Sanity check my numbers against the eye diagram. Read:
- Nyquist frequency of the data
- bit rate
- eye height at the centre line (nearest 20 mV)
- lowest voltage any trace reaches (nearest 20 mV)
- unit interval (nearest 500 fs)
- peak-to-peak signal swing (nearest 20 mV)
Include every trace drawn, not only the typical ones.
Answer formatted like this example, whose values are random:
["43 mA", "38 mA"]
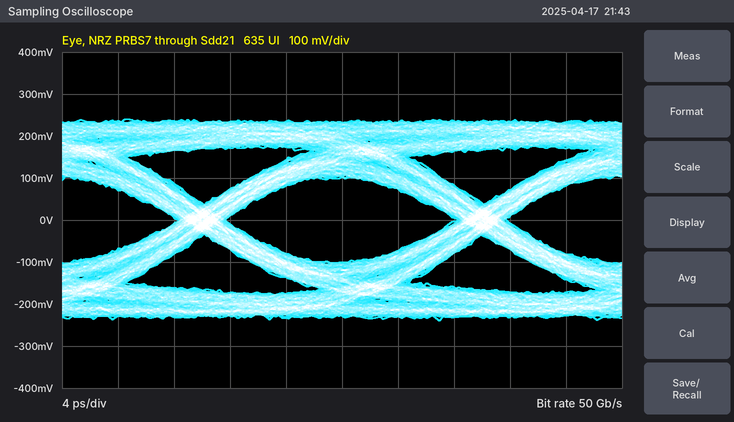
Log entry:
["25 GHz", "50 Gb/s", "200 mV", "-240 mV", "20.0 ps", "480 mV"]
